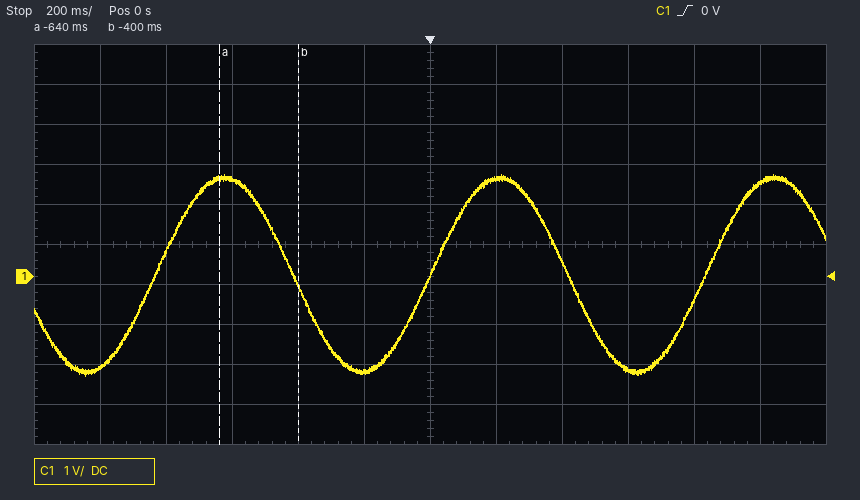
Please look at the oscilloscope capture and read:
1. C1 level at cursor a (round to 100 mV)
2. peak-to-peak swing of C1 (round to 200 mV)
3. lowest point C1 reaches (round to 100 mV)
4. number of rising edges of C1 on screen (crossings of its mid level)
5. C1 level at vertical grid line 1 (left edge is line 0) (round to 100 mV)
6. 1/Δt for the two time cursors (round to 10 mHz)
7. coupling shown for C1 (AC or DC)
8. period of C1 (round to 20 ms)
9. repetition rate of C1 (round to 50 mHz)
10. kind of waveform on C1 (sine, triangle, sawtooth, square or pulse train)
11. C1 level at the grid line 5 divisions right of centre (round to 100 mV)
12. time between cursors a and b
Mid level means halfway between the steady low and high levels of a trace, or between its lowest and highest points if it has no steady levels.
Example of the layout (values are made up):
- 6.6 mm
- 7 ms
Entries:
- 2.5 V
- 5.0 V
- -2.5 V
- 3
- -2.3 V
- 4.17 Hz
- DC
- 840 ms
- 1.20 Hz
- sine
- 2.3 V
- 240 ms
